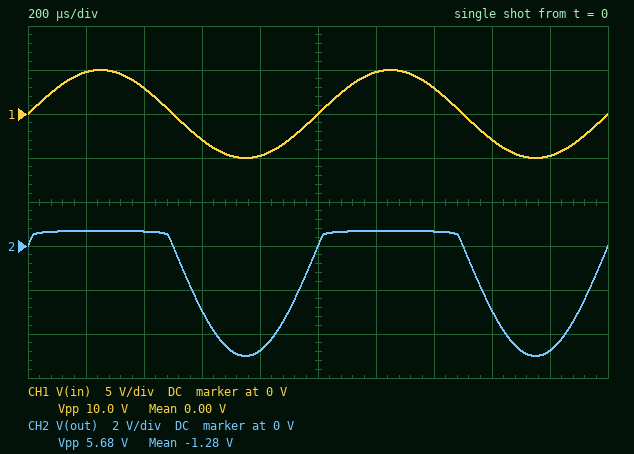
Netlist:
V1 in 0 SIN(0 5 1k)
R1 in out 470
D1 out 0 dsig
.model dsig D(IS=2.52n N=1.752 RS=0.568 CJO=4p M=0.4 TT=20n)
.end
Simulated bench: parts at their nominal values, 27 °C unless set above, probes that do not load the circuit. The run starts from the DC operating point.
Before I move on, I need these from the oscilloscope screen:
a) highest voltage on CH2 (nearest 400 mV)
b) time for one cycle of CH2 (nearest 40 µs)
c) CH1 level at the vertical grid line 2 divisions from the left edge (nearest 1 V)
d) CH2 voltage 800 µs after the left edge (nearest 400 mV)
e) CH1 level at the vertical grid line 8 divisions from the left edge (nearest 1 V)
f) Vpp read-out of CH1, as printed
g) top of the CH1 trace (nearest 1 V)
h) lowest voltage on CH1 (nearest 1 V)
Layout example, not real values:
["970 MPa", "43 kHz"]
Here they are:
["800 mV", "1.00 ms", "3 V", "-4.8 V", "-3 V", "10.0 V", "5 V", "-5 V"]
